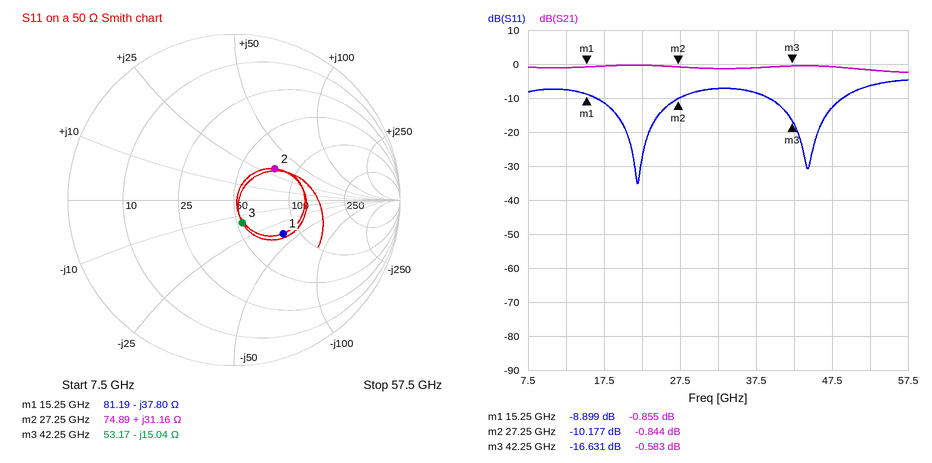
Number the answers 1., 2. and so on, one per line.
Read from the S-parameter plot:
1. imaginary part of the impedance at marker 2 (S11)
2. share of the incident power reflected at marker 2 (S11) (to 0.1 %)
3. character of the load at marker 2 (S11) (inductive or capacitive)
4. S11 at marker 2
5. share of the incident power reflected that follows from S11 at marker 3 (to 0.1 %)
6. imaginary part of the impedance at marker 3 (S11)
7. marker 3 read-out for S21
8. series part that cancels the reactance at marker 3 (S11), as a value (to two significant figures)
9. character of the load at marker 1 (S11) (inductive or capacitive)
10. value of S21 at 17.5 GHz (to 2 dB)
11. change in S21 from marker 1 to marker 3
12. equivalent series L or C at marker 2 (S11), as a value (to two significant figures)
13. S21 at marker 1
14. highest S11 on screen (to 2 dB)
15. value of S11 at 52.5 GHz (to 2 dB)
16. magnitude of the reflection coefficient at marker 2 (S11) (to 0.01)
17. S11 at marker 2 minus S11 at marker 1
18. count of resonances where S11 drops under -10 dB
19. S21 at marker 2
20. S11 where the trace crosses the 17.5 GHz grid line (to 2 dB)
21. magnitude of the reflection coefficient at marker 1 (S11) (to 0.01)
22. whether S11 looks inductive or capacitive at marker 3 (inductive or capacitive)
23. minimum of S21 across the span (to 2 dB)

1. +31.16 Ω
2. 9.6 %
3. inductive
4. -10.177 dB
5. 2.2 %
6. -15.04 Ω
7. -0.583 dB
8. 57 pH
9. capacitive
10. 0 dB
11. 0.272 dB
12. 180 pH
13. -0.855 dB
14. -4 dB
15. -6 dB
16. 0.31
17. -1.278 dB
18. 2
19. -0.844 dB
20. -12 dB
21. 0.36
22. capacitive
23. -2 dB
